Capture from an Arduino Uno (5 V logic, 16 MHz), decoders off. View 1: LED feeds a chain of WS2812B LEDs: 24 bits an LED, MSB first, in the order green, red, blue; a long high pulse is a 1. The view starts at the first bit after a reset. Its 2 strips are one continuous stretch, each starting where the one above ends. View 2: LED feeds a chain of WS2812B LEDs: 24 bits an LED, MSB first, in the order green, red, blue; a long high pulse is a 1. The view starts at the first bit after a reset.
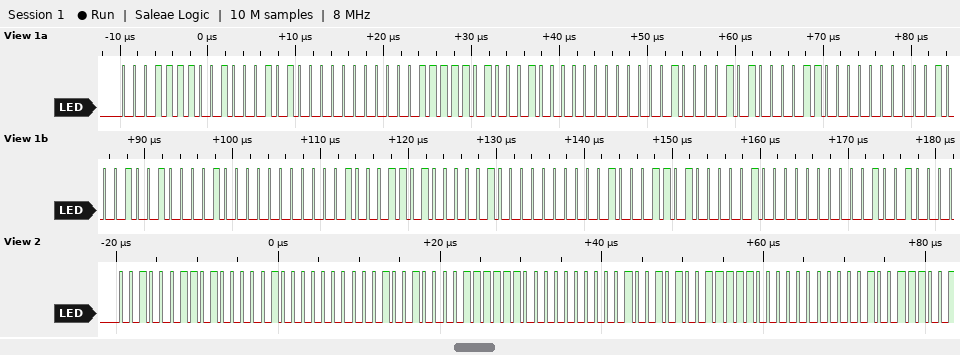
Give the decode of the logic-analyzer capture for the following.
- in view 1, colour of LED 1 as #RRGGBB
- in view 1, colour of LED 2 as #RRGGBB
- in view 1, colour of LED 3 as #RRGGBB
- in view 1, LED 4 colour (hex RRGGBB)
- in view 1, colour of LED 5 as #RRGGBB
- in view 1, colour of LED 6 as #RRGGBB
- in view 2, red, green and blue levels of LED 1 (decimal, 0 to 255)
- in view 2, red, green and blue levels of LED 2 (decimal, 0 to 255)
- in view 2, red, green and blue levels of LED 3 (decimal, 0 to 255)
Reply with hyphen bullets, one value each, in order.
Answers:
- #451E00
- #441F00
- #432100
- #422200
- #412300
- #412300
- 65, 35, 0
- 63, 36, 0
- 62, 37, 0
